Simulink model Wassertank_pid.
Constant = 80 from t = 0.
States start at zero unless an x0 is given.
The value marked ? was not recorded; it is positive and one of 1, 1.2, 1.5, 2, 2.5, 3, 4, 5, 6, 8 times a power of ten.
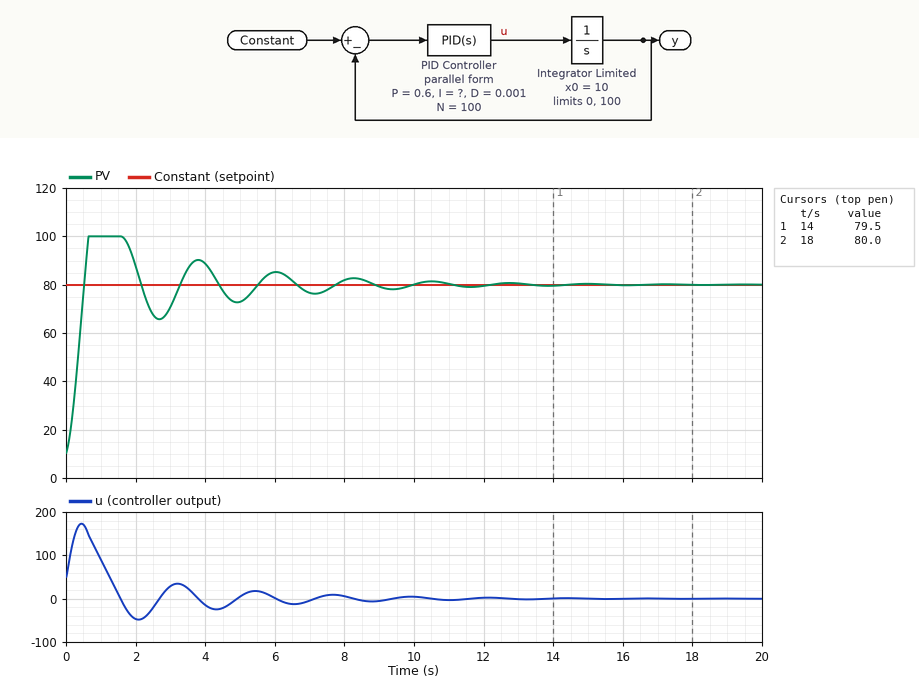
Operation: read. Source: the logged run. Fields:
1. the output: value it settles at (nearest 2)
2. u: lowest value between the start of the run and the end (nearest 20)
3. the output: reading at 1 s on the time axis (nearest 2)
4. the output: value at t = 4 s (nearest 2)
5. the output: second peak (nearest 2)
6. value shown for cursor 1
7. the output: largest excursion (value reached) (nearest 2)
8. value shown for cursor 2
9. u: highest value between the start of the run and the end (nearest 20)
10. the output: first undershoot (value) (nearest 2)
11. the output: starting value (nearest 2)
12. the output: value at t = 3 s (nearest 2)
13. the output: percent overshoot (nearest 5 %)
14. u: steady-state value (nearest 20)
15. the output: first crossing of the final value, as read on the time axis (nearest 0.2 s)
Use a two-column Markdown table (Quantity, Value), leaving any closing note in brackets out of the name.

| Quantity | Value |
|---|---|
| the output: value it settles at | 80 |
| u: lowest value between the start of the run and the end | -40 |
| the output: reading at 1 s on the time axis | 100 |
| the output: value at t = 4 s | 88 |
| the output: second peak | 90 |
| value shown for cursor 1 | 79.5 |
| the output: largest excursion (value reached) | 100 |
| value shown for cursor 2 | 80.0 |
| u: highest value between the start of the run and the end | 180 |
| the output: first undershoot (value) | 66 |
| the output: starting value | 10 |
| the output: value at t = 3 s | 70 |
| the output: percent overshoot | 30 % |
| u: steady-state value | 0 |
| the output: first crossing of the final value, as read on the time axis | 0.6 s |
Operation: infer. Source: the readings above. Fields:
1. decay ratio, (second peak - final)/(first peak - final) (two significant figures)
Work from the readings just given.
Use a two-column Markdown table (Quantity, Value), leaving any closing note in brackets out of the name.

| Quantity | Value |
|---|---|
| decay ratio, (second peak - final)/(first peak - final) | 0.50 |
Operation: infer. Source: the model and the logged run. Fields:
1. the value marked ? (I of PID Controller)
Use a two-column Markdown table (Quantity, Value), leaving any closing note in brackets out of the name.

| Quantity | Value |
|---|---|
| the value marked ? | 8 |
